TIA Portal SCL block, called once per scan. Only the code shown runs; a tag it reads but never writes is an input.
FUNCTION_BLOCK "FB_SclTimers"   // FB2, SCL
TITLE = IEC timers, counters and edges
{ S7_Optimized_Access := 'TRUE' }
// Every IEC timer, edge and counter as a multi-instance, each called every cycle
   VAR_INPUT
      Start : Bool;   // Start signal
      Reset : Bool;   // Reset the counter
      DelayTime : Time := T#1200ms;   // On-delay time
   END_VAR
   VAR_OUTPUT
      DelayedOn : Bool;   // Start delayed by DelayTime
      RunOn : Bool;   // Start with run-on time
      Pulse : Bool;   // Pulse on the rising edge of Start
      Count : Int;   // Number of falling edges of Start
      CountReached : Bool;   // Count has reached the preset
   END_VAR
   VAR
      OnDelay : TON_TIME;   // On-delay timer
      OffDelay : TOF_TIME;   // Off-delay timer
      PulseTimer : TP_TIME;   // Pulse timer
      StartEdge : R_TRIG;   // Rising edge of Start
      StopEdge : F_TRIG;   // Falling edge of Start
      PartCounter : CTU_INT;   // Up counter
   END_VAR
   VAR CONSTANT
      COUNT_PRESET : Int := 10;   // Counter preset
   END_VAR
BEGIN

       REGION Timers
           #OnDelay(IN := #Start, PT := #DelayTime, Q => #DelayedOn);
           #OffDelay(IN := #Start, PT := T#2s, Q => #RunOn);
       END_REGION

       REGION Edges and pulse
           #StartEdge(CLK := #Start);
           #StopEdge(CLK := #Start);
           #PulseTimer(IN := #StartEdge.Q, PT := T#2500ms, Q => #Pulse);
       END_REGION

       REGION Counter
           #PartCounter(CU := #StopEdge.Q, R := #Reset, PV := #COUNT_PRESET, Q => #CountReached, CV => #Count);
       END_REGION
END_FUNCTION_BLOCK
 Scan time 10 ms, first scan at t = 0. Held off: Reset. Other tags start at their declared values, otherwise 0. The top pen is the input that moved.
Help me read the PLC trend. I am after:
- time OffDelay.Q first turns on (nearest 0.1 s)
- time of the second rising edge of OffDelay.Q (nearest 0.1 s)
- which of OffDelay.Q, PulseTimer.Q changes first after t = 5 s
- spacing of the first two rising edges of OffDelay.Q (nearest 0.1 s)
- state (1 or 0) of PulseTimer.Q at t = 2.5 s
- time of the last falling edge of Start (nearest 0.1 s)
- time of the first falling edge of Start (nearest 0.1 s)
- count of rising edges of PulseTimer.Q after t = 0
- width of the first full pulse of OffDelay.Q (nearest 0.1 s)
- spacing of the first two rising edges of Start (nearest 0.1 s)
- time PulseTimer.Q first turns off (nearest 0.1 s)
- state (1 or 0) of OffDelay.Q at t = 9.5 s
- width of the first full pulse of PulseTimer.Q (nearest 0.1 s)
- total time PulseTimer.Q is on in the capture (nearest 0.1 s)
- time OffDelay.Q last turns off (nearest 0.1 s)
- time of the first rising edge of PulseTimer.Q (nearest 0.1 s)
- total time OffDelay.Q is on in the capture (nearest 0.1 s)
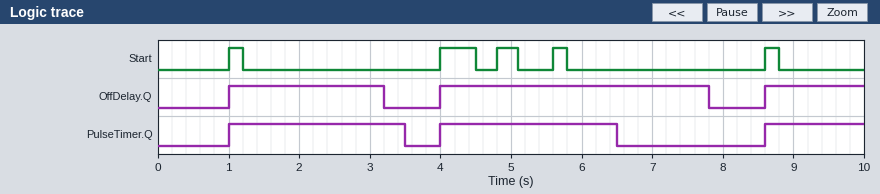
1.0 s
4.0 s
PulseTimer.Q
3.0 s
1
8.8 s
1.2 s
3
2.2 s
3.0 s
3.5 s
1
2.5 s
6.4 s
7.8 s
1.0 s
7.4 s
